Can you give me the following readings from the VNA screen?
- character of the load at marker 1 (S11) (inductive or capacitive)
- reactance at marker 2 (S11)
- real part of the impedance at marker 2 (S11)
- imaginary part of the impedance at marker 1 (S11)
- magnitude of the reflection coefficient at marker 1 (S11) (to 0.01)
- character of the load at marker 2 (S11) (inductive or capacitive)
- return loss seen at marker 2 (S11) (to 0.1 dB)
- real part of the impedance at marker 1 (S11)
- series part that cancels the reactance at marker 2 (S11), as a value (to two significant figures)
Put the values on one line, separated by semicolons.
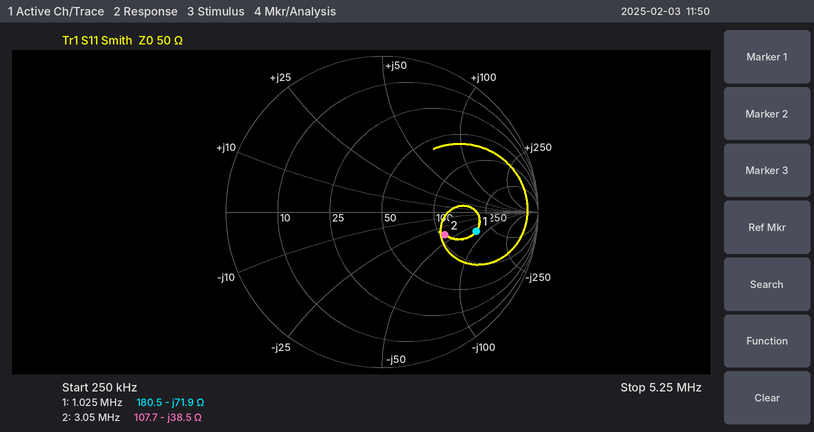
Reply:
capacitive; -38.5 Ω; 107.7 Ω; -71.9 Ω; 0.62; capacitive; 7.4 dB; 180.5 Ω; 2.0 µH
